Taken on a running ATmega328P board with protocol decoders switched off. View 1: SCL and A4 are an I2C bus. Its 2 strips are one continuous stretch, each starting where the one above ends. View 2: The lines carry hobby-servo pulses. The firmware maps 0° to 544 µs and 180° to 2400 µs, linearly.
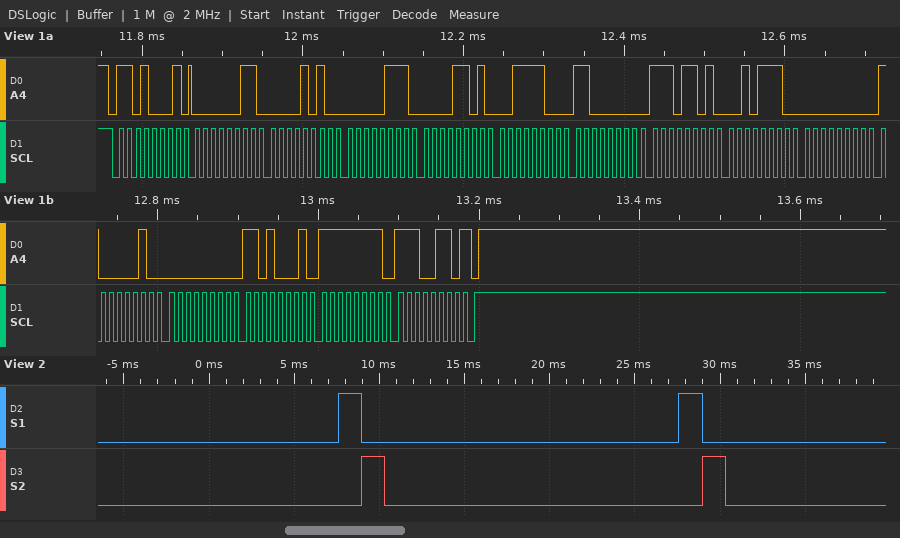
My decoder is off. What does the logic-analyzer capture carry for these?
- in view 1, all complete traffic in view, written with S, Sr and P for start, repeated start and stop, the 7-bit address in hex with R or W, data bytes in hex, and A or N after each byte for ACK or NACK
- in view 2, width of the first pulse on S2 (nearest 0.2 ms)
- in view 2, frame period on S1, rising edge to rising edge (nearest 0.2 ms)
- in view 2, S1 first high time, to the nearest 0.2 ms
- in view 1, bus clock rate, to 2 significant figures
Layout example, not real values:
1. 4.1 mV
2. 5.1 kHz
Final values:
1. S 68R A 03 A 0A A 07 A 0D A 3C A C0 A ED A 2E A 00 A 82 A 00 A D1 A FF A E6 N P
2. 1.4 ms
3. 20.0 ms
4. 1.4 ms
5. 100 kHz
